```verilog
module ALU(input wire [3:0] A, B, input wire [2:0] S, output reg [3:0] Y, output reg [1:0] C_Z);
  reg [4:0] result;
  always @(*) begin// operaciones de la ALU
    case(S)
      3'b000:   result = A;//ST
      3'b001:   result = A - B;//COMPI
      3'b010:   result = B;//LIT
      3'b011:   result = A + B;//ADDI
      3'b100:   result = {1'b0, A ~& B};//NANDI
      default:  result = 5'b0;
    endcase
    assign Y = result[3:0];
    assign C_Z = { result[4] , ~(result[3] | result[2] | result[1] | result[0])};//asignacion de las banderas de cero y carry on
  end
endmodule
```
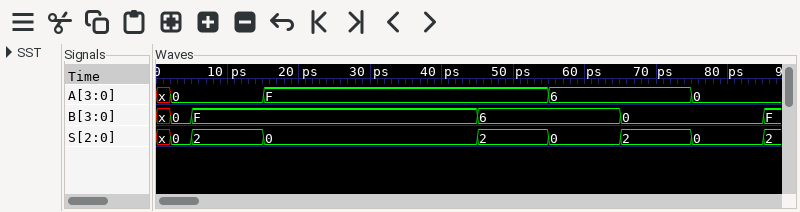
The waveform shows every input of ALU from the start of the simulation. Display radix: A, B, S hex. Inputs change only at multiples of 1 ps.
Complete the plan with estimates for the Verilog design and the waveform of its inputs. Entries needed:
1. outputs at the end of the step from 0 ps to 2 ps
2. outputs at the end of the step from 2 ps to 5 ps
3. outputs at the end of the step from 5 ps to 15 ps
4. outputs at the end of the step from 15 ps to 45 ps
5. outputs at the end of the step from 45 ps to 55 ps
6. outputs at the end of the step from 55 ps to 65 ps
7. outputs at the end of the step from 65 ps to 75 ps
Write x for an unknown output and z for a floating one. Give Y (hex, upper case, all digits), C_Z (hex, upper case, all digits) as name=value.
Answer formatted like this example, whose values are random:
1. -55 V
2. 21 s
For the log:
1. Y=x, C_Z=x
2. Y=0, C_Z=1
3. Y=F, C_Z=0
4. Y=F, C_Z=0
5. Y=6, C_Z=0
6. Y=6, C_Z=0
7. Y=0, C_Z=1
